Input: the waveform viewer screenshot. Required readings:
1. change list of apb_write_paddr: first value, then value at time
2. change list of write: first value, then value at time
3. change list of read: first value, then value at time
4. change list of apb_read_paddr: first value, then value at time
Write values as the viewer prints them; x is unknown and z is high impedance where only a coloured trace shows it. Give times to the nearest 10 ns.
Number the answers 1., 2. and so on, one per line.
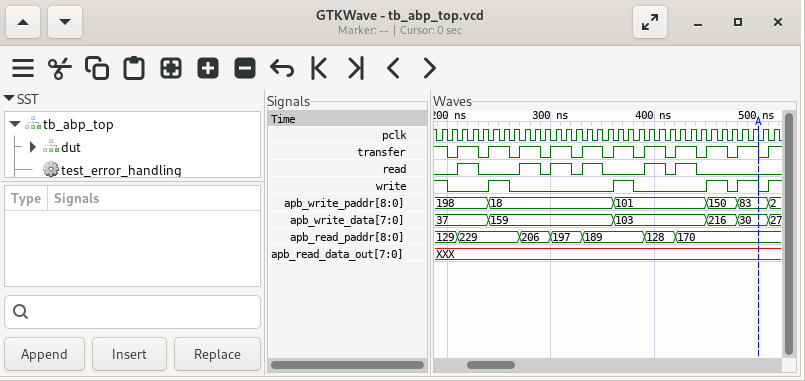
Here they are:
1. 198, 18 at 240 ns, 101 at 360 ns, 150 at 450 ns, 83 at 480 ns, 2 at 510 ns
2. 1, 0 at 200 ns, 1 at 240 ns, 0 at 260 ns, 1 at 360 ns, 0 at 380 ns, 1 at 450 ns, 0 at 470 ns, 1 at 480 ns, 0 at 500 ns, 1 at 510 ns
3. 0, 1 at 210 ns, 0 at 230 ns, 1 at 270 ns, 0 at 290 ns, 1 at 300 ns, 0 at 320 ns, 1 at 330 ns, 0 at 350 ns, 1 at 390 ns, 0 at 410 ns, 1 at 420 ns, 0 at 440 ns
4. 129, 229 at 210 ns, 206 at 270 ns, 197 at 300 ns, 189 at 330 ns, 128 at 390 ns, 170 at 420 ns
